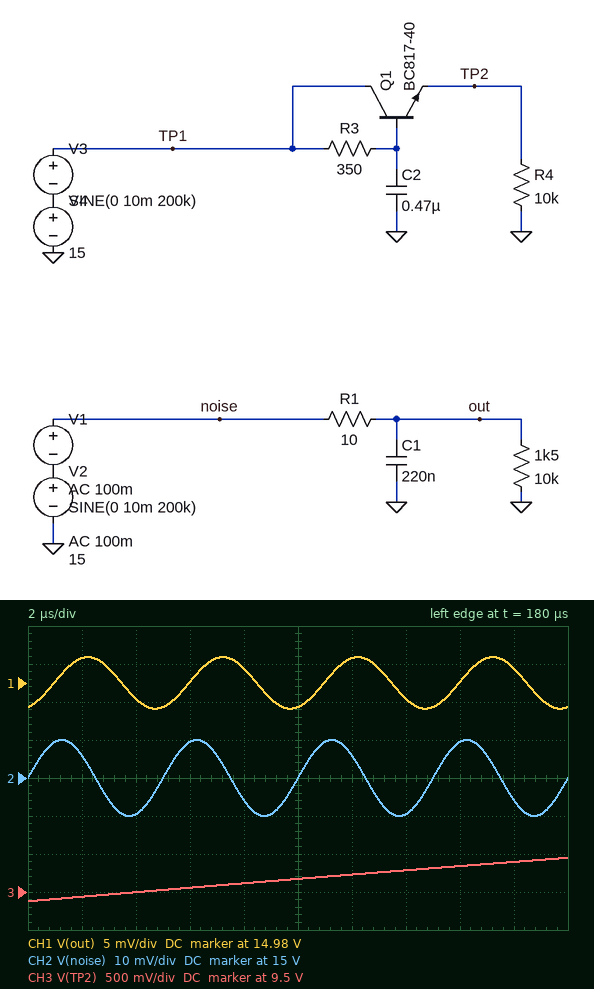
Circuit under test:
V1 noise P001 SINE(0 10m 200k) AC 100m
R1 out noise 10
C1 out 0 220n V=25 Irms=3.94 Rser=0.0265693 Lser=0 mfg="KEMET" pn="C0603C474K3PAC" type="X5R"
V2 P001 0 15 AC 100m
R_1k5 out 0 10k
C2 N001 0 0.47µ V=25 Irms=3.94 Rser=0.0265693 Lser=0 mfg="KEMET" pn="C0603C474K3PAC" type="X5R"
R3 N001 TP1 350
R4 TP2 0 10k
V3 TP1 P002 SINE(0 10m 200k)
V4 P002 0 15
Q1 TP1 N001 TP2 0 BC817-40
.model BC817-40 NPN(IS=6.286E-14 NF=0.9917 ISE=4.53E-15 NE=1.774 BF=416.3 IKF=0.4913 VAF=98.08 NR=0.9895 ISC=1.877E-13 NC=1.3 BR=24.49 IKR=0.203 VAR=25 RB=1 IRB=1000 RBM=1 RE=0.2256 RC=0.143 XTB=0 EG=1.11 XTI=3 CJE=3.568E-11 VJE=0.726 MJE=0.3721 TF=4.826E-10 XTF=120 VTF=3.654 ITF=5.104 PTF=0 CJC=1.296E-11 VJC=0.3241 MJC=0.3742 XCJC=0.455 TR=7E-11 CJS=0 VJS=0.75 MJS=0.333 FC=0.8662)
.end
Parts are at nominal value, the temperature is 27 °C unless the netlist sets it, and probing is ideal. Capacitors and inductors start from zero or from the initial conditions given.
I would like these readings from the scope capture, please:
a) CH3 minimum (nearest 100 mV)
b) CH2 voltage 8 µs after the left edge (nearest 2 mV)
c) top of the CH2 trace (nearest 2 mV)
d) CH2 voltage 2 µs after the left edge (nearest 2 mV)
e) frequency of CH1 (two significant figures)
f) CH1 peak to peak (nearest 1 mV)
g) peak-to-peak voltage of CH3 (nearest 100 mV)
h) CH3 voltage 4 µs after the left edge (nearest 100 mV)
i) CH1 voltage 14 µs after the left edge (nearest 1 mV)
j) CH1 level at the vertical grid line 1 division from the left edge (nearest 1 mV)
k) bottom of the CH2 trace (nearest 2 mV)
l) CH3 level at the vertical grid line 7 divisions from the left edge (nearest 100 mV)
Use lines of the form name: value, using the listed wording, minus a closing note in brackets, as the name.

CH3 minimum: 9.4 V
CH2 voltage 8 µs after the left edge: 14.994 V
top of the CH2 trace: 15.010 V
CH2 voltage 2 µs after the left edge: 15.006 V
frequency of CH1: 200 kHz
CH1 peak to peak: 7 mV
peak-to-peak voltage of CH3: 600 mV
CH3 voltage 4 µs after the left edge: 9.5 V
CH1 voltage 14 µs after the left edge: 14.983 V
CH1 level at the vertical grid line 1 division from the left edge: 14.988 V
bottom of the CH2 trace: 14.990 V
CH3 level at the vertical grid line 7 divisions from the left edge: 9.8 V
